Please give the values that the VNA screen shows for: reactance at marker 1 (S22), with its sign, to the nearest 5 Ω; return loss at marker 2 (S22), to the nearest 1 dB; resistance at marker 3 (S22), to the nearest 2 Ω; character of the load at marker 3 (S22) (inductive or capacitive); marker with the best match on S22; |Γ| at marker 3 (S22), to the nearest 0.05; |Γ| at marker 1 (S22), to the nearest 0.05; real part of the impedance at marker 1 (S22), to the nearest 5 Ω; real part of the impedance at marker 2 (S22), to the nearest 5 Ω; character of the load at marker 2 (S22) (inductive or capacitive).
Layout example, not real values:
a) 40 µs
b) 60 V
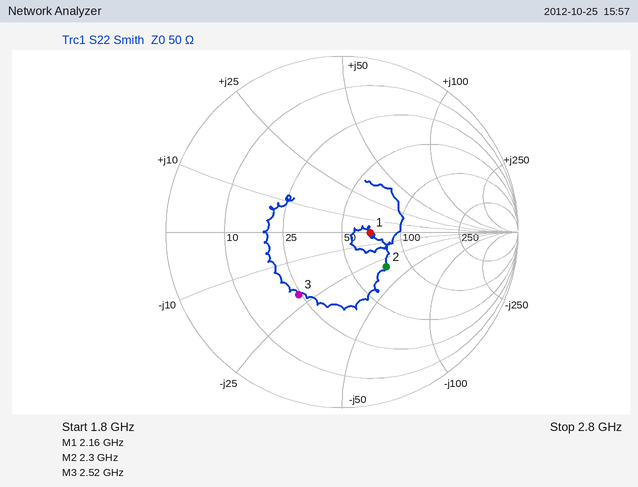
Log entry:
a) 0 Ω
b) 10 dB
c) 24 Ω
d) capacitive
e) marker 1
f) 0.45
g) 0.15
h) 70 Ω
i) 75 Ω
j) capacitive
